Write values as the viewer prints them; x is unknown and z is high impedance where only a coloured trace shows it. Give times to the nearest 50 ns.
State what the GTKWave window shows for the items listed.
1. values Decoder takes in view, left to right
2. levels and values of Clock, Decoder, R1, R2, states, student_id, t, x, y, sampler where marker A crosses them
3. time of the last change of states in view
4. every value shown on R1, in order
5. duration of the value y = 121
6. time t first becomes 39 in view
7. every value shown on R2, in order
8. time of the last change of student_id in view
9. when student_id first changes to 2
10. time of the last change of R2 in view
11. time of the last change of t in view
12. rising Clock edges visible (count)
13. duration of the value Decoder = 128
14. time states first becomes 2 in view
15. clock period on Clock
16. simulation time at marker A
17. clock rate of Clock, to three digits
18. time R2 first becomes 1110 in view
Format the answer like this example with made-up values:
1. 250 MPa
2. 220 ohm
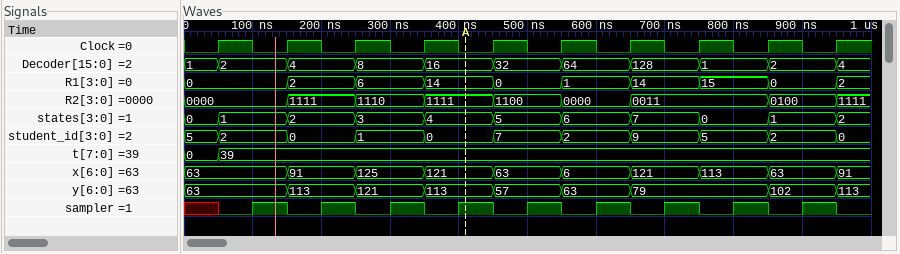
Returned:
1. 1, 2, 4, 8, 16, 32, 64, 128, 1, 2, 4
2. Clock=0, Decoder=16, R1=14, R2=1111, states=4, student_id=0, t=39, x=121, y=113, sampler=1
3. 950 ns
4. 0, 2, 6, 14, 0, 1, 14, 15, 0, 2
5. 100 ns
6. 50 ns
7. 0000, 1111, 1110, 1111, 1100, 0000, 0011, 0100, 1111
8. 950 ns
9. 50 ns
10. 950 ns
11. 50 ns
12. 10
13. 100 ns
14. 150 ns
15. 100 ns
16. 400 ns
17. 10.0 MHz
18. 250 ns
